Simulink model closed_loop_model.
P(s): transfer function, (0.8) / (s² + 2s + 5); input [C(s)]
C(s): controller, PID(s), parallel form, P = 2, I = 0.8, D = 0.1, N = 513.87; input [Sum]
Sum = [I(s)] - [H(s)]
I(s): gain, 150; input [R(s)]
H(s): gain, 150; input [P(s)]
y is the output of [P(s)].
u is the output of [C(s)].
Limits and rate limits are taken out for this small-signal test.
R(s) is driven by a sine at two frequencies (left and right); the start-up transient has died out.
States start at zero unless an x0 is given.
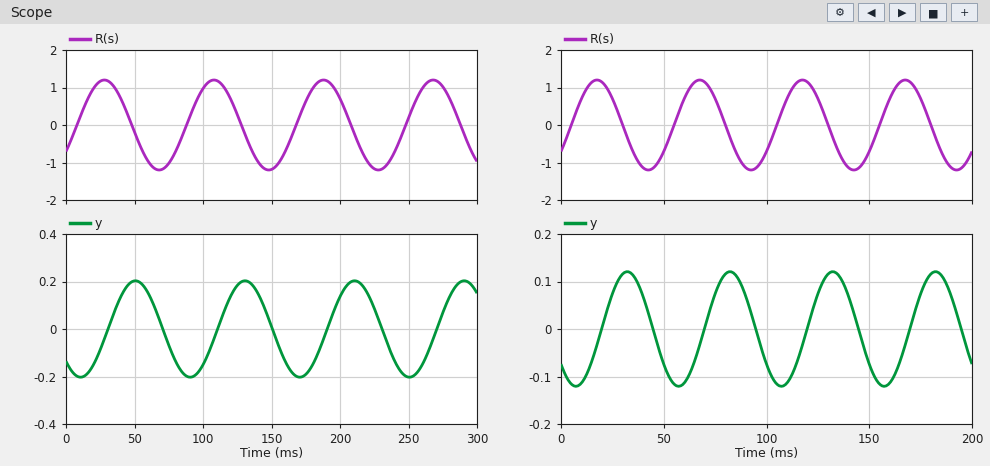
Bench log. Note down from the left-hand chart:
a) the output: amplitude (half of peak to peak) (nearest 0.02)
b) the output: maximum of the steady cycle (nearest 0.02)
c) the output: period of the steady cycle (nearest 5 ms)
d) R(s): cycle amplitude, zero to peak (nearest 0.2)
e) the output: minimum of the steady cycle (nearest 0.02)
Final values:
0.20
0.20
80 ms
1.2
-0.20
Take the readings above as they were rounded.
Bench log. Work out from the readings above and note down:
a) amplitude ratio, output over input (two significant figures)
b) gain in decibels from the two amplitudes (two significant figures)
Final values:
0.17
-16 dB
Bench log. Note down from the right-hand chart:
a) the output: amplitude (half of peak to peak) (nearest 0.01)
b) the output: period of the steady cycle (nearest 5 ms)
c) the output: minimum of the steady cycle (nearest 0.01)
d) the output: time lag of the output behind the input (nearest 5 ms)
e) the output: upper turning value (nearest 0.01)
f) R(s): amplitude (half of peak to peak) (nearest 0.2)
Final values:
0.12
50 ms
-0.12
15 ms
0.12
1.2
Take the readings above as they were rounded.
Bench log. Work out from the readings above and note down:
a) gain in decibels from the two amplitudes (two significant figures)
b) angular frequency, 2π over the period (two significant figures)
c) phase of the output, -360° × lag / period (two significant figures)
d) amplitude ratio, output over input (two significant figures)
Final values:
-20 dB
0.13 rad/ms
-110°
0.10
